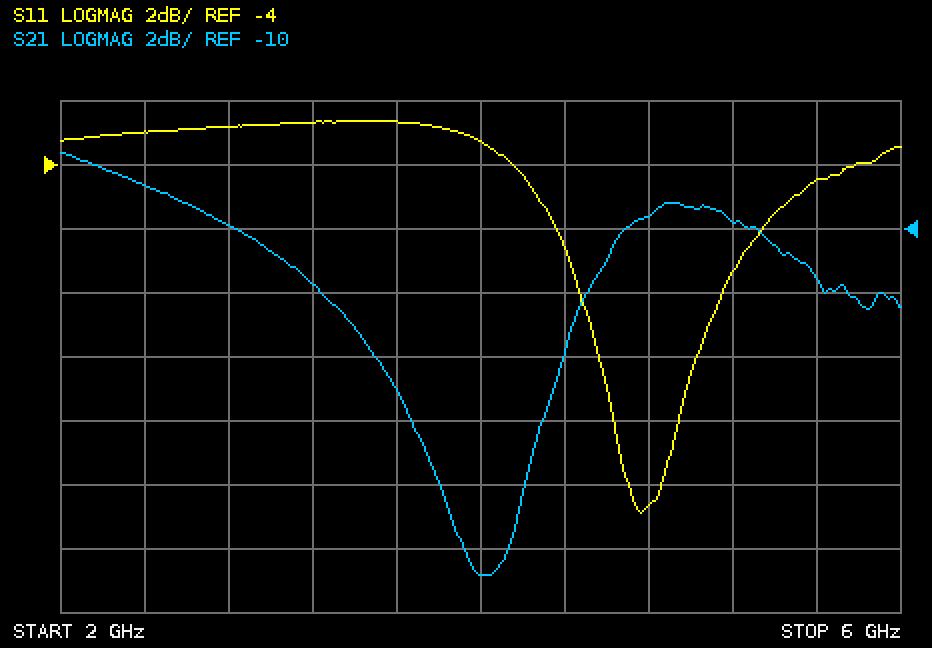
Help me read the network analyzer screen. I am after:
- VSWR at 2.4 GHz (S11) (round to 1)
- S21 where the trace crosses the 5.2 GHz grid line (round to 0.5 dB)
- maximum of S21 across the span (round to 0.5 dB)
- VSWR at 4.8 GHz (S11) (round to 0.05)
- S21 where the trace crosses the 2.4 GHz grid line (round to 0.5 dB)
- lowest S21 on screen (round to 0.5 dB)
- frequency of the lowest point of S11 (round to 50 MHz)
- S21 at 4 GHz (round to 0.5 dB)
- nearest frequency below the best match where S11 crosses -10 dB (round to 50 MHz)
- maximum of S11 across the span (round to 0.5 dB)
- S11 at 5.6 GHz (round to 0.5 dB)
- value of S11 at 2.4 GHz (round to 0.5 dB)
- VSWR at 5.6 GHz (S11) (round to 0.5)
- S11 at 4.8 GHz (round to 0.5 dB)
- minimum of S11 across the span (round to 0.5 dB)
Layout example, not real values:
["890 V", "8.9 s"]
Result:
["6", "-10.0 dB", "-7.5 dB", "1.45", "-8.5 dB", "-21.0 dB", "4.75 GHz", "-21.0 dB", "4.55 GHz", "-2.5 dB", "-4.5 dB", "-3.0 dB", "4.0", "-14.5 dB", "-15.0 dB"]
